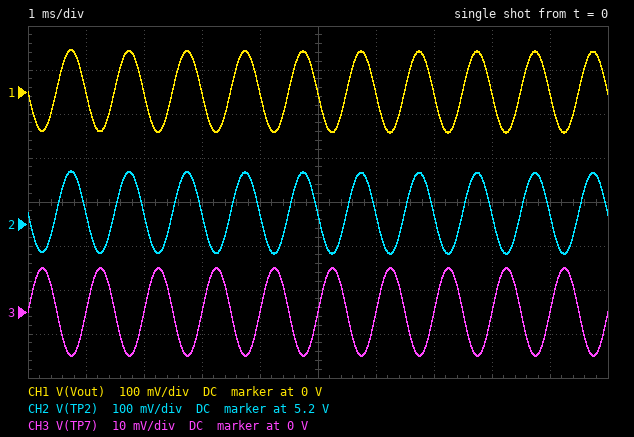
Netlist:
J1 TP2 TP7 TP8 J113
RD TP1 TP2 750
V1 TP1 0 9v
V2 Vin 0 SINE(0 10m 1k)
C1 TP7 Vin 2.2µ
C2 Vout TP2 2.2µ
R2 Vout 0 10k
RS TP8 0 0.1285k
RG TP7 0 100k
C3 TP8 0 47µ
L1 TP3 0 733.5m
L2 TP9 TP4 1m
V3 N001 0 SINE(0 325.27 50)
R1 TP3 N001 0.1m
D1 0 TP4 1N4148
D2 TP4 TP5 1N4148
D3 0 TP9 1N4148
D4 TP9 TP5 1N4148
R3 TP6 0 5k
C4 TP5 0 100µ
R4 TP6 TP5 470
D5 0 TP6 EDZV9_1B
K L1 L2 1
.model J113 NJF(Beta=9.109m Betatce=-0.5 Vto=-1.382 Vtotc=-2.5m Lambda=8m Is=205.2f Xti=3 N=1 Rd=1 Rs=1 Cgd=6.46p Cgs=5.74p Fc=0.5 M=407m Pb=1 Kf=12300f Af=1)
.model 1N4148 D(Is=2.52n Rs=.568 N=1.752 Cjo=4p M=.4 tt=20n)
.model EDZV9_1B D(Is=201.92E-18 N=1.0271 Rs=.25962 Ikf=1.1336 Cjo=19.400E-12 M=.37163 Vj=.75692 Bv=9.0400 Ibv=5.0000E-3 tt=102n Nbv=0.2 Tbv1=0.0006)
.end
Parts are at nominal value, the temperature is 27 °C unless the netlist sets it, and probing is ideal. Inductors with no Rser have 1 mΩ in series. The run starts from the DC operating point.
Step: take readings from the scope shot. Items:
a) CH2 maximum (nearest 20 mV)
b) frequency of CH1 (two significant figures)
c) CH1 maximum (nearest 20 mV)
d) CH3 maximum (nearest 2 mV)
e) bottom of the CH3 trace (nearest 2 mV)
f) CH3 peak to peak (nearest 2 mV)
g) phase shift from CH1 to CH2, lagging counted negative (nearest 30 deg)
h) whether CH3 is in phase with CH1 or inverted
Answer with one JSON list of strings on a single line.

["5.32 V", "1.0 kHz", "100 mV", "10 mV", "-10 mV", "20 mV", "0 deg", "inverted"]
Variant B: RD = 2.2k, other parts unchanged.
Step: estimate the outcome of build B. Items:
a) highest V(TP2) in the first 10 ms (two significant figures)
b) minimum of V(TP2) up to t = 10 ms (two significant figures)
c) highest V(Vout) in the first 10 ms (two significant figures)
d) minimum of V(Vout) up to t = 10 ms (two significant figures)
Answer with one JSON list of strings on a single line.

["760 mV", "750 mV", "4.2 mV", "-4.0 mV"]
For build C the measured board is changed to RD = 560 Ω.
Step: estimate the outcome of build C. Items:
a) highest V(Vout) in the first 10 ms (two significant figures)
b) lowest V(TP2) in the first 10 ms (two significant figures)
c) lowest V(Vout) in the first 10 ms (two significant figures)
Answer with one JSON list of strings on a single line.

["73 mV", "6.1 V", "-71 mV"]
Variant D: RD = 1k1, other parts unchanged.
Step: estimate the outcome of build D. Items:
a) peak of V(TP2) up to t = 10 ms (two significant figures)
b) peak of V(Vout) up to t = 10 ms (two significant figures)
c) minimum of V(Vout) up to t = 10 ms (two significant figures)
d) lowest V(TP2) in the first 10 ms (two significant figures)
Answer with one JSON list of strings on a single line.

["3.6 V", "130 mV", "-130 mV", "3.4 V"]
